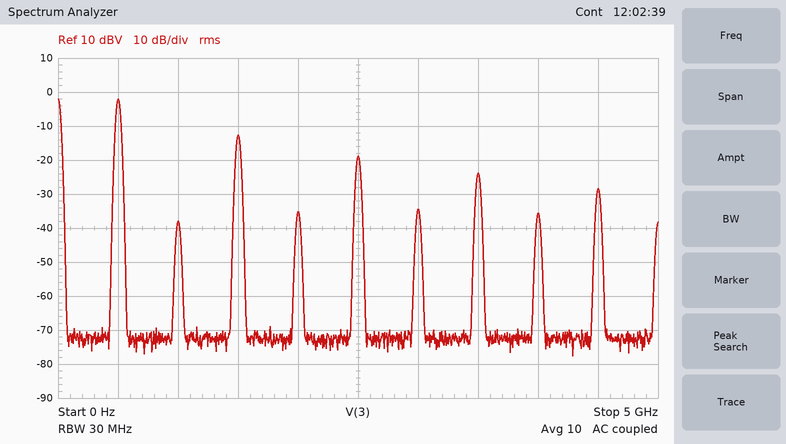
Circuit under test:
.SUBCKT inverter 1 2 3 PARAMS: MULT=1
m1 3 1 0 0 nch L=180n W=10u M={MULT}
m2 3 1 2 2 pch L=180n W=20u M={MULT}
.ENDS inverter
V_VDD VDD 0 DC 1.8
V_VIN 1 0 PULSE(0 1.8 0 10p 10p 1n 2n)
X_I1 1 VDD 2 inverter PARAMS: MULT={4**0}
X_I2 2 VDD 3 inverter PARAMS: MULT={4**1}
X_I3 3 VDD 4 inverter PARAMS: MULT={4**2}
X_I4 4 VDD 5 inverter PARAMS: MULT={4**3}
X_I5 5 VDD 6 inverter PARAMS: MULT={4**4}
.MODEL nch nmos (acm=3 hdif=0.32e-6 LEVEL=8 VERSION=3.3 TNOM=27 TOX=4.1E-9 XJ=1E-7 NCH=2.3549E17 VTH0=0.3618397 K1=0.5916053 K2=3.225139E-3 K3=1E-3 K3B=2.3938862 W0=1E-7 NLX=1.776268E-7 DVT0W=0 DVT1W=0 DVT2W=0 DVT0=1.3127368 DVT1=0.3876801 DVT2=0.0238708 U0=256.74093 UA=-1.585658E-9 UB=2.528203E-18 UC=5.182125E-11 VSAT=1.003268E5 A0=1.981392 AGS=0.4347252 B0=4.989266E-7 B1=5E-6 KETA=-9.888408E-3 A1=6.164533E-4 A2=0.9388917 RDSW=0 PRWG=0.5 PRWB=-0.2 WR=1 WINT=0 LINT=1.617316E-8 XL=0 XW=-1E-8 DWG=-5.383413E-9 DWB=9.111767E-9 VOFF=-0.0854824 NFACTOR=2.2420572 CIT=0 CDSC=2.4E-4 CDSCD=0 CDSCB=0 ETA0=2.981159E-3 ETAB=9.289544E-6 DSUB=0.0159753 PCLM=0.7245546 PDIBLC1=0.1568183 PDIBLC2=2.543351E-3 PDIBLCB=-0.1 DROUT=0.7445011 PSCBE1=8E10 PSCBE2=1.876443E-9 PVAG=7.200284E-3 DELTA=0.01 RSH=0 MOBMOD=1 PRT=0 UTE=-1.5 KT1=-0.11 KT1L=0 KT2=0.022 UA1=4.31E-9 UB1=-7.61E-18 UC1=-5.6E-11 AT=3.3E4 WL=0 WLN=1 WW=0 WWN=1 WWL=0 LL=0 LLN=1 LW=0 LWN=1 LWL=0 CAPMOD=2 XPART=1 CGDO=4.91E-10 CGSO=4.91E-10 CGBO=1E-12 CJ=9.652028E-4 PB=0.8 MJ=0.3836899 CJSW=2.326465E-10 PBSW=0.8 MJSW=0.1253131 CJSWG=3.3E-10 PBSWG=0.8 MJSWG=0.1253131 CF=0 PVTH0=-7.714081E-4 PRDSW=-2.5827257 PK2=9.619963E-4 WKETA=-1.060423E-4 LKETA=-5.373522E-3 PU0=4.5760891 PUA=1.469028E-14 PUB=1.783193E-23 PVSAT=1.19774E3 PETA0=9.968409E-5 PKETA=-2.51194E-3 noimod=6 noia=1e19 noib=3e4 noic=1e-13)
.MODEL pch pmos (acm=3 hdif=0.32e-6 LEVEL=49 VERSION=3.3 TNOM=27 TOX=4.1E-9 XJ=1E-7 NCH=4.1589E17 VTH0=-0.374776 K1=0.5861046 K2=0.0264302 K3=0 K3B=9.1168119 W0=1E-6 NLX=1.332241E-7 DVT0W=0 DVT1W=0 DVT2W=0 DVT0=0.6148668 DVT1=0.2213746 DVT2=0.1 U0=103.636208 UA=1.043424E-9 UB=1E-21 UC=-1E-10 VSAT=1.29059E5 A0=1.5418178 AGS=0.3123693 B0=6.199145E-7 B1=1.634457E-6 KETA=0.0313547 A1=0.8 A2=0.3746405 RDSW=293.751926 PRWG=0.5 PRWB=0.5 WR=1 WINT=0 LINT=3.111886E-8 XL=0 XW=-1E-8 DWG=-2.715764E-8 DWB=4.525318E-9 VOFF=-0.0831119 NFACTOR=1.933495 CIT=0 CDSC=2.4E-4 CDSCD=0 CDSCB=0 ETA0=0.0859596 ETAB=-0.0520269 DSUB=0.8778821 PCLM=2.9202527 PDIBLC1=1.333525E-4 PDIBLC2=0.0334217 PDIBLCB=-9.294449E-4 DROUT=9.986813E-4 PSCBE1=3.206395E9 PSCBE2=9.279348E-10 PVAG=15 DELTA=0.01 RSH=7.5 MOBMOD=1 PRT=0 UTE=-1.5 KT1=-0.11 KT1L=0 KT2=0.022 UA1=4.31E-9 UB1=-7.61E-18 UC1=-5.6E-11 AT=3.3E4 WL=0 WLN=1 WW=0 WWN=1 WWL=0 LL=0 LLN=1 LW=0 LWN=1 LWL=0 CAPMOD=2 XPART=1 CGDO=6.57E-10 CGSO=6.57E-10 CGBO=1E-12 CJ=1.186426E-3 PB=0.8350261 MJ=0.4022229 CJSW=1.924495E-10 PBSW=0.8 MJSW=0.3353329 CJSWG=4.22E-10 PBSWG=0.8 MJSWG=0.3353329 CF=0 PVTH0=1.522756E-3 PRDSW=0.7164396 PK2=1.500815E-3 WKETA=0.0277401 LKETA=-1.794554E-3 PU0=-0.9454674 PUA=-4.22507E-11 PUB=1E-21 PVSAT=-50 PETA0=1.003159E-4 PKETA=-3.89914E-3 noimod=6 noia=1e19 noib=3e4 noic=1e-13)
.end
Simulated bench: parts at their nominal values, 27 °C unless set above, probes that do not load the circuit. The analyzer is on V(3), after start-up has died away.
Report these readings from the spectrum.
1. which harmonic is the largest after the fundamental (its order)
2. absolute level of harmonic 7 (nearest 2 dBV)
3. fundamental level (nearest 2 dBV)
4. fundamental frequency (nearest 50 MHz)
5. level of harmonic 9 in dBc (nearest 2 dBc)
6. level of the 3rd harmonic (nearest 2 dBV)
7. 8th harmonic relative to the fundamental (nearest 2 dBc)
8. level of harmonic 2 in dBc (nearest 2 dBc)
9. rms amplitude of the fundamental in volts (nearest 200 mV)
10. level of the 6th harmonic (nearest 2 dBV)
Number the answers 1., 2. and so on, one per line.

1. 3
2. -24 dBV
3. -2 dBV
4. 500 MHz
5. -26 dBc
6. -12 dBV
7. -34 dBc
8. -36 dBc
9. 800 mV
10. -34 dBV
